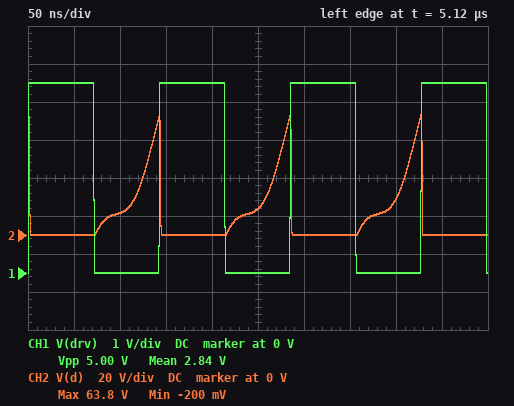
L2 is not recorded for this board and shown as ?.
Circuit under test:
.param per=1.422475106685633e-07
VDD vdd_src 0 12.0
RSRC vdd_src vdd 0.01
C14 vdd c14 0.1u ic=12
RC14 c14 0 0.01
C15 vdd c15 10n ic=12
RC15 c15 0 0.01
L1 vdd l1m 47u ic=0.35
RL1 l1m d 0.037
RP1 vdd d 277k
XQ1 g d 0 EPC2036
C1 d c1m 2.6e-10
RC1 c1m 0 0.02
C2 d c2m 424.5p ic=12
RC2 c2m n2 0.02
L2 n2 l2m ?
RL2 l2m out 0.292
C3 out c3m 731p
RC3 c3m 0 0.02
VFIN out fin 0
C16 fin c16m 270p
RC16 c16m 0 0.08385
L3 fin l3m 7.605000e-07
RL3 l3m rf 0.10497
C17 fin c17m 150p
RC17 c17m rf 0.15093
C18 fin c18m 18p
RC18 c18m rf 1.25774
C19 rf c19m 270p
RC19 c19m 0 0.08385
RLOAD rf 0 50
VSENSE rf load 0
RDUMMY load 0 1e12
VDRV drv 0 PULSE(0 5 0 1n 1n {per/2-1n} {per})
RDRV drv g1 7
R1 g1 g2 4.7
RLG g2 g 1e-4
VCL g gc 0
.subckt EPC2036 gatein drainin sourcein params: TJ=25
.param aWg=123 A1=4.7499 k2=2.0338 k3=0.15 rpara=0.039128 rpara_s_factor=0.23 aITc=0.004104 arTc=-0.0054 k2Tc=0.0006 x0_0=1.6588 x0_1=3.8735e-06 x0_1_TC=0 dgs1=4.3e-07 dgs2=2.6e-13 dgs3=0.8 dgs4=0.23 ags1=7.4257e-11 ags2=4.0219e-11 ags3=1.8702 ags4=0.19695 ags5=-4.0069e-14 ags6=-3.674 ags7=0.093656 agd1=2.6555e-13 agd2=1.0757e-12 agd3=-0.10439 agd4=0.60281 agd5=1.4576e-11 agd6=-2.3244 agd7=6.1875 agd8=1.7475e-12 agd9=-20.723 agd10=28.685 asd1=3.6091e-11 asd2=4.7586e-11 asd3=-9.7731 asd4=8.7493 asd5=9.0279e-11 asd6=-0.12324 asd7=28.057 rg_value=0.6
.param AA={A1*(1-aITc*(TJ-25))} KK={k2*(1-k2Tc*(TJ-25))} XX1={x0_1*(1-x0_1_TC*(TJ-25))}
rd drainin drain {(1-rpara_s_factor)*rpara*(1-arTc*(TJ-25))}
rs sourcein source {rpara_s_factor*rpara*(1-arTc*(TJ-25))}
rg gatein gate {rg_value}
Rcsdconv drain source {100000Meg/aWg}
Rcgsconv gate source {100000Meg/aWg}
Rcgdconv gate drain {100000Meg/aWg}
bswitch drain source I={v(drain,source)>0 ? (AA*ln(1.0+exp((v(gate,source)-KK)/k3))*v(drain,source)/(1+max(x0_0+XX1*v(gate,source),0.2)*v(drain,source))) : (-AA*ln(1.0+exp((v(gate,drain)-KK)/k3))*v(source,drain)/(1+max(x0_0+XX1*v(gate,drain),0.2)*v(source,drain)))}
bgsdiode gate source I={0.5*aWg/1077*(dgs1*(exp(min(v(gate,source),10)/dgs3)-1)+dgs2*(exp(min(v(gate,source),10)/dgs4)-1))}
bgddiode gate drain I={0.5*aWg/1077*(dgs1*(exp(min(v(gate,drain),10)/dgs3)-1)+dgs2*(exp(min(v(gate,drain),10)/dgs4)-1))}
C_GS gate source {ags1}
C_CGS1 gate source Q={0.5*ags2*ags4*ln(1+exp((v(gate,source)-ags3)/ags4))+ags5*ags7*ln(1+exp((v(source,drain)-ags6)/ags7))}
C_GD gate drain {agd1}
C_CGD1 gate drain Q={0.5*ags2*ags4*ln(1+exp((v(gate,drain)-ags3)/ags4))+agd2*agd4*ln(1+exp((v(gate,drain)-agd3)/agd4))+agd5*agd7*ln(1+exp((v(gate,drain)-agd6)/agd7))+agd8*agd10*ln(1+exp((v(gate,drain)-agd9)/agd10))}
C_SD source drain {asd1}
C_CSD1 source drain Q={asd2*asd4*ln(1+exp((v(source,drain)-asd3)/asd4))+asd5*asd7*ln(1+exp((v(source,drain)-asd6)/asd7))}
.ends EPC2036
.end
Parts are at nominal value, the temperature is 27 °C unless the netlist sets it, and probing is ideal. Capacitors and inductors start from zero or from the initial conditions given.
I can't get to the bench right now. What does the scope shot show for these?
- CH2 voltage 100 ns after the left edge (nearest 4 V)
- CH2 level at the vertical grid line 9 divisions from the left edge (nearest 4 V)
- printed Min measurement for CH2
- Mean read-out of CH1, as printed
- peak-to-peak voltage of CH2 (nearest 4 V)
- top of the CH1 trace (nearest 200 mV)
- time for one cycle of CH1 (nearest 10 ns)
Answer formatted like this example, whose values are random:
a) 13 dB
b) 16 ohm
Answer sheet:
a) 12 V
b) 0 V
c) -200 mV
d) 2.84 V
e) 64 V
f) 5.0 V
g) 140 ns
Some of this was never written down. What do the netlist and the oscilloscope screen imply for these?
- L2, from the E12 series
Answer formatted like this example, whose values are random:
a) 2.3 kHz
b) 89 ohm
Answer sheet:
a) 1.2 µH
